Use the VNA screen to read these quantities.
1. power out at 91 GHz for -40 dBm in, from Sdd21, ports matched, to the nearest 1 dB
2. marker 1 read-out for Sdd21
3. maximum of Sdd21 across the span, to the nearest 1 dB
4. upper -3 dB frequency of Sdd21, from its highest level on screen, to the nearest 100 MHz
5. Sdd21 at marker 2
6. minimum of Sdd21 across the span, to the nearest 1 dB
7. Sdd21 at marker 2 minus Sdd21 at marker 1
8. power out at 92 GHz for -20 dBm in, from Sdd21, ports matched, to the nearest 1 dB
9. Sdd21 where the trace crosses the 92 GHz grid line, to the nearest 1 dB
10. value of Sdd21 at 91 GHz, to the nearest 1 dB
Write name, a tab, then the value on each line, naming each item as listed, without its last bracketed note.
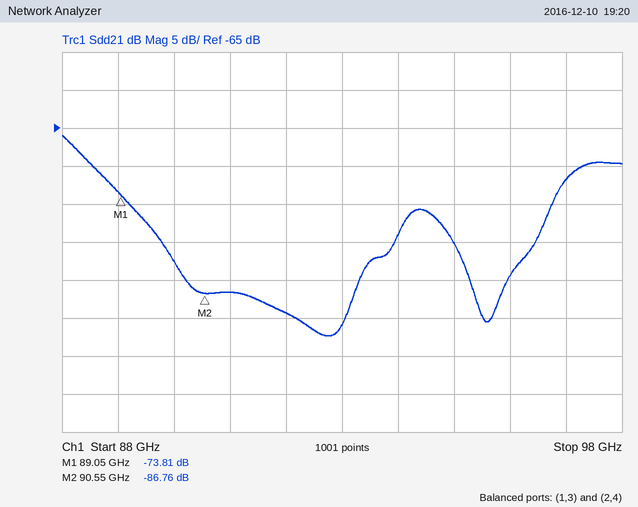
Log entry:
power out at 91 GHz for -40 dBm in, from Sdd21, ports matched, to the nearest 1 dB	-127 dBm
marker 1 read-out for Sdd21	-73.81 dB
maximum of Sdd21 across the span, to the nearest 1 dB	-66 dB
upper -3 dB frequency of Sdd21, from its highest level on screen, to the nearest 100 MHz	88.4 GHz
Sdd21 at marker 2	-86.76 dB
minimum of Sdd21 across the span, to the nearest 1 dB	-92 dB
Sdd21 at marker 2 minus Sdd21 at marker 1	-12.95 dB
power out at 92 GHz for -20 dBm in, from Sdd21, ports matched, to the nearest 1 dB	-109 dBm
Sdd21 where the trace crosses the 92 GHz grid line, to the nearest 1 dB	-89 dB
value of Sdd21 at 91 GHz, to the nearest 1 dB	-87 dB
